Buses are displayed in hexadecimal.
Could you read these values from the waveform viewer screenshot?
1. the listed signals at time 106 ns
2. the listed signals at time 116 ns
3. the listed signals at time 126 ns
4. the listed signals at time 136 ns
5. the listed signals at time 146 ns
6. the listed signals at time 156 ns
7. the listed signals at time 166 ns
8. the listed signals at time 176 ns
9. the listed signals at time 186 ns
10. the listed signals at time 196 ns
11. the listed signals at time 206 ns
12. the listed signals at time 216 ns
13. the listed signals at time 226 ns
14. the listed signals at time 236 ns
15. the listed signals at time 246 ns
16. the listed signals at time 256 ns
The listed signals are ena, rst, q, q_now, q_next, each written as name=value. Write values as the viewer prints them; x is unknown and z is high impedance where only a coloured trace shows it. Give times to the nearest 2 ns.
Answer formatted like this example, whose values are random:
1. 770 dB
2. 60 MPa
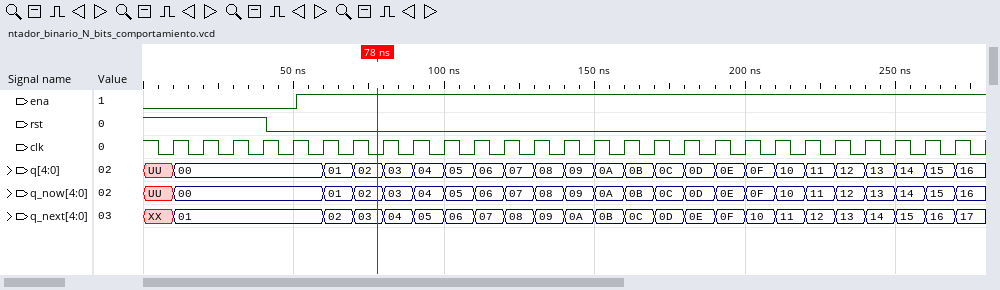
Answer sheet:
1. ena=1, rst=0, q=05, q_now=05, q_next=06
2. ena=1, rst=0, q=06, q_now=06, q_next=07
3. ena=1, rst=0, q=07, q_now=07, q_next=08
4. ena=1, rst=0, q=08, q_now=08, q_next=09
5. ena=1, rst=0, q=09, q_now=09, q_next=0A
6. ena=1, rst=0, q=0A, q_now=0A, q_next=0B
7. ena=1, rst=0, q=0B, q_now=0B, q_next=0C
8. ena=1, rst=0, q=0C, q_now=0C, q_next=0D
9. ena=1, rst=0, q=0D, q_now=0D, q_next=0E
10. ena=1, rst=0, q=0E, q_now=0E, q_next=0F
11. ena=1, rst=0, q=0F, q_now=0F, q_next=10
12. ena=1, rst=0, q=10, q_now=10, q_next=11
13. ena=1, rst=0, q=11, q_now=11, q_next=12
14. ena=1, rst=0, q=12, q_now=12, q_next=13
15. ena=1, rst=0, q=13, q_now=13, q_next=14
16. ena=1, rst=0, q=14, q_now=14, q_next=15
